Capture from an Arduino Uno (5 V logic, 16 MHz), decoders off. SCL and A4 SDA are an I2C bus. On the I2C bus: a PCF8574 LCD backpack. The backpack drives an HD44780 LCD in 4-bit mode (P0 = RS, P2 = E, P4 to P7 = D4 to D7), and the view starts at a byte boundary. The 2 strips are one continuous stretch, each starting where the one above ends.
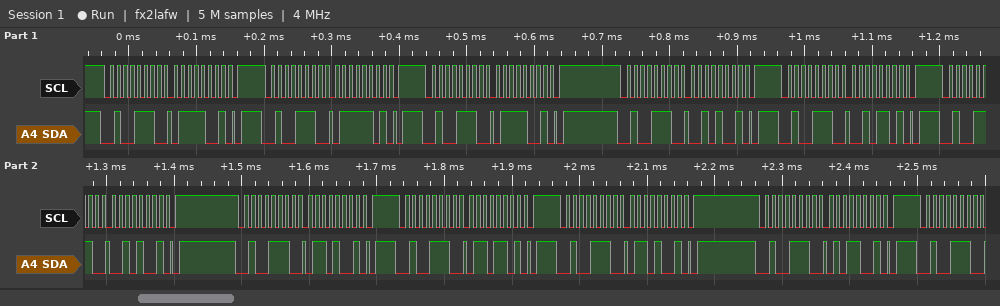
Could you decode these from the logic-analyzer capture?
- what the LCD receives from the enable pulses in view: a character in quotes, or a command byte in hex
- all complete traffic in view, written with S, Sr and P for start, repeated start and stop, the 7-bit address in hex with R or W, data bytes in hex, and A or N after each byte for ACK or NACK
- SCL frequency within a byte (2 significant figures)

'r'
S 27W A 79 A P S 27W A 7D A P S 27W A 79 A P S 27W A 29 A P S 27W A 2D A P S 27W A 29 A P S 27W A 69 A P S 27W A 6D A P S 27W A 69 A P S 27W A 59 A P S 27W A
100 kHz
